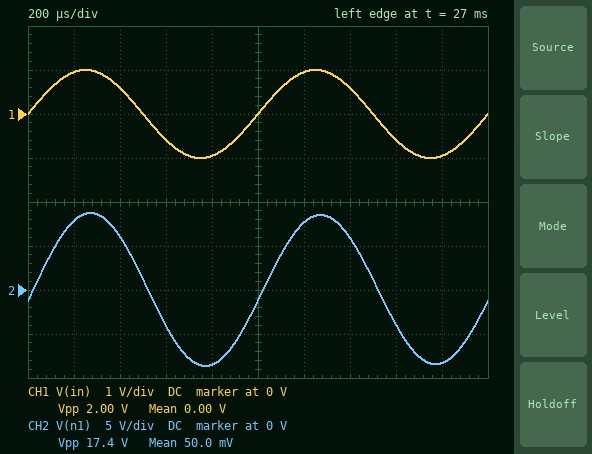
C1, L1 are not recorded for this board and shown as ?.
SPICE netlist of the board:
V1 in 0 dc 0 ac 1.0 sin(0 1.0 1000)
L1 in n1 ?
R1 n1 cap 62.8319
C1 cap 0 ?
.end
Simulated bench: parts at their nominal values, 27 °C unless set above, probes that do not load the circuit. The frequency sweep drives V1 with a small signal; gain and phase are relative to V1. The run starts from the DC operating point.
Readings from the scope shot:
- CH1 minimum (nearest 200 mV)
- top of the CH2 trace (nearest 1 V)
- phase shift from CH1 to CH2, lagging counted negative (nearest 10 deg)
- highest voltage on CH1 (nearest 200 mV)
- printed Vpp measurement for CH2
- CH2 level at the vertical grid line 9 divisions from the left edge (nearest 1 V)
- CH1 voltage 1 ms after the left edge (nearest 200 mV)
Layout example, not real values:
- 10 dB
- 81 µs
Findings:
- -1.0 V
- 9 V
- -10 deg
- 1.0 V
- 17.4 V
- -8 V
- 0 V
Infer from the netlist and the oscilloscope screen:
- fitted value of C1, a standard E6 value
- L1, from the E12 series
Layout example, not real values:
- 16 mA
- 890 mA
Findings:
- 68 nF
- 330 mH
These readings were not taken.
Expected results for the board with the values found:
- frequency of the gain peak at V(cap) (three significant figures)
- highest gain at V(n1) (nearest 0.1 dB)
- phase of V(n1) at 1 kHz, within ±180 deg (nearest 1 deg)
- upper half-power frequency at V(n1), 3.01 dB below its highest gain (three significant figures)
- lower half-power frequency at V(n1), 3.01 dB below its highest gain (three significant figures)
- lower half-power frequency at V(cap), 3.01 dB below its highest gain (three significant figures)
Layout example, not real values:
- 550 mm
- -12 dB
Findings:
- 1.06 kHz
- 30.9 dB
- -12 deg
- 1.08 kHz
- 1.05 kHz
- 1.05 kHz
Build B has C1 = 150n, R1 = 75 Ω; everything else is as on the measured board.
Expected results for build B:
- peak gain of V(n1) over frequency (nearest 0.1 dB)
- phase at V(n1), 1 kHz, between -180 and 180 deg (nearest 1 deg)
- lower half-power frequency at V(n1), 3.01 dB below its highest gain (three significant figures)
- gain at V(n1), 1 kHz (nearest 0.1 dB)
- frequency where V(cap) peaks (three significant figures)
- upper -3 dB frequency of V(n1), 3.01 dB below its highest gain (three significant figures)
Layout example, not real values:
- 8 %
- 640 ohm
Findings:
- 25.9 dB
- -172 deg
- 697 Hz
- 0.4 dB
- 715 Hz
- 733 Hz
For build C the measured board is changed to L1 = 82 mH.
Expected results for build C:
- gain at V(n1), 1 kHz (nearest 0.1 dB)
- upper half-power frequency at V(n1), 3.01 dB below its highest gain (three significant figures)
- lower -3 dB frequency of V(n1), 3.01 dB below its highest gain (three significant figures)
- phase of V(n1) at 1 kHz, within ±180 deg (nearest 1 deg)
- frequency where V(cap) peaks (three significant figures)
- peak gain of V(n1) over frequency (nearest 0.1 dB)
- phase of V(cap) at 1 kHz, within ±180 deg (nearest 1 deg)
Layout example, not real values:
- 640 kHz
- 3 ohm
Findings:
- 2.2 dB
- 2.19 kHz
- 2.07 kHz
- 0 deg
- 2.13 kHz
- 24.9 dB
- -2 deg
